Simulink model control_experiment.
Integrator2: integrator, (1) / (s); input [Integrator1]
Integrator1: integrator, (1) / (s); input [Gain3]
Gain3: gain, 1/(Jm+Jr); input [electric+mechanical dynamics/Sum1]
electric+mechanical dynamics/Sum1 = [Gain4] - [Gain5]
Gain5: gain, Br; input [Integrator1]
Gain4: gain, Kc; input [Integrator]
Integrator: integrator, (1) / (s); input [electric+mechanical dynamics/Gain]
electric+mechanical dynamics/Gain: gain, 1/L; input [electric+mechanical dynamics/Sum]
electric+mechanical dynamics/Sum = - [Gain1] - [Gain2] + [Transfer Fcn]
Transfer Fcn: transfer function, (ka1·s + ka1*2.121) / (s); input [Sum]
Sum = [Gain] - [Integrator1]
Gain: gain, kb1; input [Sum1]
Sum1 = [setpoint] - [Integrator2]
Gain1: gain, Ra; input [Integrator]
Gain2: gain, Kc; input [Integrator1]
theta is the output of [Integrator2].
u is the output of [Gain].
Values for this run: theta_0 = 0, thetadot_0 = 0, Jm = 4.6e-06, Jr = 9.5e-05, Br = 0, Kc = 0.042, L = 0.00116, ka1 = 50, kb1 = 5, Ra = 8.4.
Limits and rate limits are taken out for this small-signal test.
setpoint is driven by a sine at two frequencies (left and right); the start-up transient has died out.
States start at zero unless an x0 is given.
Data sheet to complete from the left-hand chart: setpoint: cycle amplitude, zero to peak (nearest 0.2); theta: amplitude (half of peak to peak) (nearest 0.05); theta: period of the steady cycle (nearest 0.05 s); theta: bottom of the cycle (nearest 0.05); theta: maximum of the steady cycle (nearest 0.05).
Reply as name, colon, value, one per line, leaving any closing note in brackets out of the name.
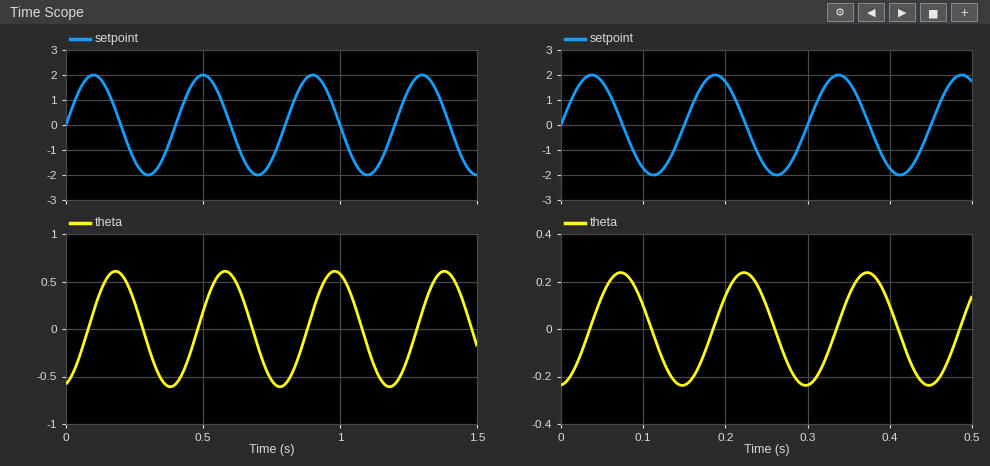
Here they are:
setpoint: cycle amplitude, zero to peak: 2.0
theta: amplitude (half of peak to peak): 0.60
theta: period of the steady cycle: 0.40 s
theta: bottom of the cycle: -0.60
theta: maximum of the steady cycle: 0.60
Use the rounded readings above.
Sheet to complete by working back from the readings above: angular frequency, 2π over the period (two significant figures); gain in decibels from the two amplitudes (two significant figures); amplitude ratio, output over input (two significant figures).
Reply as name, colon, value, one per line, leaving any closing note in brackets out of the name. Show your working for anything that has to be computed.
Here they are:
angular frequency, 2π over the period: 2π / 0.4 = 16 rad/s
gain in decibels from the two amplitudes: 20 log10(0.6 / 2) = -10 dB
amplitude ratio, output over input: 0.6 / 2 = 0.30
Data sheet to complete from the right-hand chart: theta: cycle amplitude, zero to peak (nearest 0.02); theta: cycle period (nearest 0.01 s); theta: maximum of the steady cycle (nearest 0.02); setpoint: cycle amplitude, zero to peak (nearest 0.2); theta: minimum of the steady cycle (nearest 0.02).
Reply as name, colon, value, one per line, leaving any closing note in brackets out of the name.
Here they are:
theta: cycle amplitude, zero to peak: 0.24
theta: cycle period: 0.15 s
theta: maximum of the steady cycle: 0.24
setpoint: cycle amplitude, zero to peak: 2.0
theta: minimum of the steady cycle: -0.24
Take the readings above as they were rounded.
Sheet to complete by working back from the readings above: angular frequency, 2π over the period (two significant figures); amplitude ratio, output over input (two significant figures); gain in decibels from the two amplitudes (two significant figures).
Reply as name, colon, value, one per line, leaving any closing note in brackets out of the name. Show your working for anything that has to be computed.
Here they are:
angular frequency, 2π over the period: 2π / 0.15 = 42 rad/s
amplitude ratio, output over input: 0.24 / 2 = 0.12
gain in decibels from the two amplitudes: 20 log10(0.24 / 2) = -18 dB
